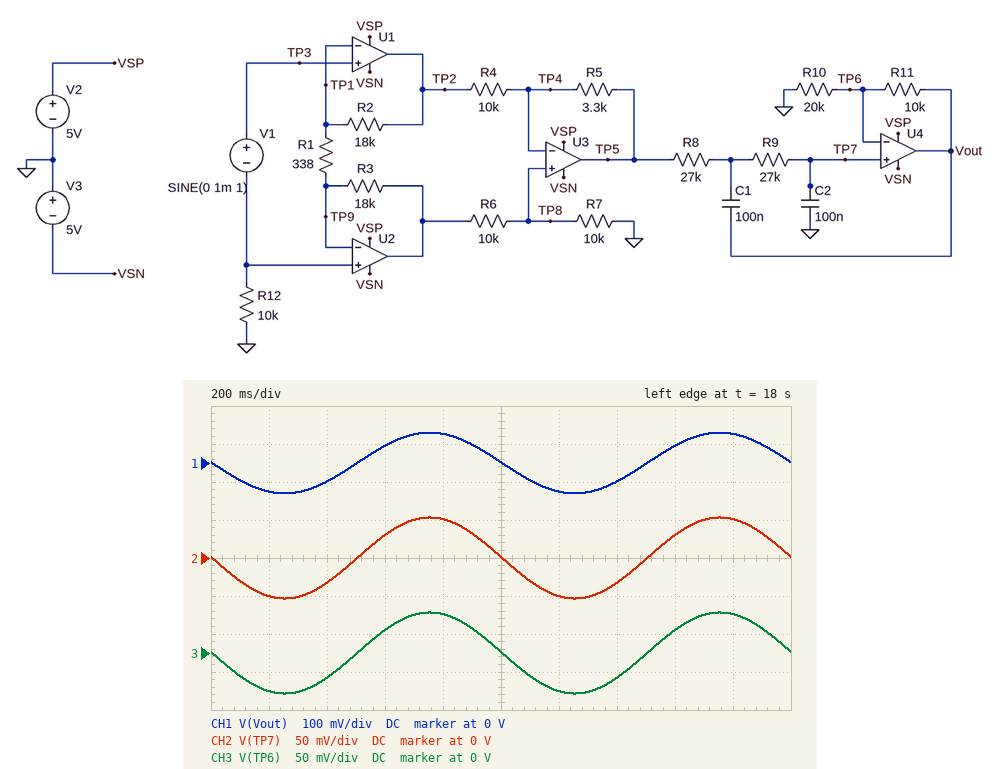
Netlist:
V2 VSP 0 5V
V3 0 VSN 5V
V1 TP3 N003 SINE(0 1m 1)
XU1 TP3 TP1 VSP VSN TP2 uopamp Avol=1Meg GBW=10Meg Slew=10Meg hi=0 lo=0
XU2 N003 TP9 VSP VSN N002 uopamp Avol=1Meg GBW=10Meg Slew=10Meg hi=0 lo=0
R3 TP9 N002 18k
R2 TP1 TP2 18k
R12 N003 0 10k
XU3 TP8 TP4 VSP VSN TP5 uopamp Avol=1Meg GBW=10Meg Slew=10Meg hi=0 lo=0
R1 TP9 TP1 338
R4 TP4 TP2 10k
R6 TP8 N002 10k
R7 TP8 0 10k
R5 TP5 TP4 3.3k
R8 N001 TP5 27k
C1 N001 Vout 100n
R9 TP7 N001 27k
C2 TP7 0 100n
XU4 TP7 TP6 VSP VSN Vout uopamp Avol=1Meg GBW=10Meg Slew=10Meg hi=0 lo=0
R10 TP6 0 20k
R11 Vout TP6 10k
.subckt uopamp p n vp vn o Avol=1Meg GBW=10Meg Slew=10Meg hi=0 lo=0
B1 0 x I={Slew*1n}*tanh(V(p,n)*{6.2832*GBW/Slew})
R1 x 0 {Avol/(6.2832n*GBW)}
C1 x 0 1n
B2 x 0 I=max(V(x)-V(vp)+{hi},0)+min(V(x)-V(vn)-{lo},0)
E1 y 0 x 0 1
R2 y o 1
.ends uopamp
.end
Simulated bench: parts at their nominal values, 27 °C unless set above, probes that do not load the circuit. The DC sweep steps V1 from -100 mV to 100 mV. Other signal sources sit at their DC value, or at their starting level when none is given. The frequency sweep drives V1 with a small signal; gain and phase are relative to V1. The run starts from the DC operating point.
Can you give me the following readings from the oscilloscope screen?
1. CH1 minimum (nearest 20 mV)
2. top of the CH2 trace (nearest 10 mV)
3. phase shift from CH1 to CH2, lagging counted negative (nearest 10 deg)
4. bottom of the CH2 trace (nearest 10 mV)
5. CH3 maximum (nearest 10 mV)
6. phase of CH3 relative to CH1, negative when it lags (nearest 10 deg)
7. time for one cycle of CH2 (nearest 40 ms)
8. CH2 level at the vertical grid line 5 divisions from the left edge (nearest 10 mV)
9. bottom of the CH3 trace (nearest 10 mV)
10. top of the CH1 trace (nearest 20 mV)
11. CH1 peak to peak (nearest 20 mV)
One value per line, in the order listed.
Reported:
-80 mV
50 mV
0 deg
-50 mV
50 mV
0 deg
1.00 s
0 V
-50 mV
80 mV
160 mV
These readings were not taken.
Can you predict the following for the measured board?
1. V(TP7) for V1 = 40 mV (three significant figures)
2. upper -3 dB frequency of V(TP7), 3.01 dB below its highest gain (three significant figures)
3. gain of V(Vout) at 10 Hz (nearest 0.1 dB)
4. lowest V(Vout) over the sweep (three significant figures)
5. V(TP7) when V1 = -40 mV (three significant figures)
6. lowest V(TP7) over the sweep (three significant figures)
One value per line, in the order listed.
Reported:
-2.13 V
55.4 Hz
38.0 dB
-5.01 V
2.13 V
-4.91 V
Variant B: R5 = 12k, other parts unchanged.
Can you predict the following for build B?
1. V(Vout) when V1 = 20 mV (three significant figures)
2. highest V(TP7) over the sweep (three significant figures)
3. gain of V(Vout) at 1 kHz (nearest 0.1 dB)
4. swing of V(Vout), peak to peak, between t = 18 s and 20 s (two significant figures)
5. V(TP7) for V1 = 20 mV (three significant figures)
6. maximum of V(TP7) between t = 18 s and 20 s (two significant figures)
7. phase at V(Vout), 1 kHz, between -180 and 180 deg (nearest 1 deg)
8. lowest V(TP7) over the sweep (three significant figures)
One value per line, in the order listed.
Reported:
-3.71 V
5.01 V
-3.8 dB
370 mV
-2.47 V
120 mV
4 deg
-5.01 V
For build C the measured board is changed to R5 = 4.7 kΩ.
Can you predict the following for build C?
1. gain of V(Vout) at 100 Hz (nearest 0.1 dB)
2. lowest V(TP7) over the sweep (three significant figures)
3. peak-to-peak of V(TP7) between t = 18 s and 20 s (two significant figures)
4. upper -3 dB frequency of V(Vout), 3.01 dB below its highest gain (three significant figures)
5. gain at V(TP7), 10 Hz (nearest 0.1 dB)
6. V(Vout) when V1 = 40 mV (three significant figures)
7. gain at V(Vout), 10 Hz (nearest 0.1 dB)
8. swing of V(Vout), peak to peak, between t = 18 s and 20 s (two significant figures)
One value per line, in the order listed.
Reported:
29.7 dB
-5.01 V
130 mV
55.4 Hz
36.2 dB
-3.88 V
39.7 dB
190 mV
